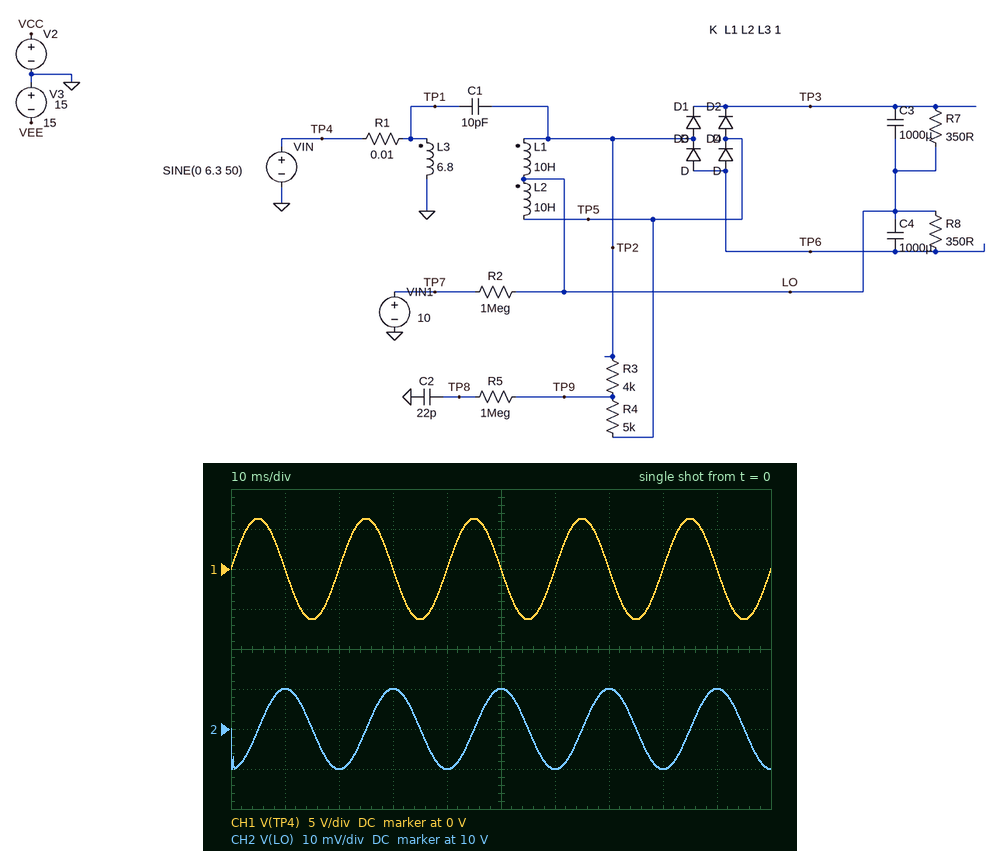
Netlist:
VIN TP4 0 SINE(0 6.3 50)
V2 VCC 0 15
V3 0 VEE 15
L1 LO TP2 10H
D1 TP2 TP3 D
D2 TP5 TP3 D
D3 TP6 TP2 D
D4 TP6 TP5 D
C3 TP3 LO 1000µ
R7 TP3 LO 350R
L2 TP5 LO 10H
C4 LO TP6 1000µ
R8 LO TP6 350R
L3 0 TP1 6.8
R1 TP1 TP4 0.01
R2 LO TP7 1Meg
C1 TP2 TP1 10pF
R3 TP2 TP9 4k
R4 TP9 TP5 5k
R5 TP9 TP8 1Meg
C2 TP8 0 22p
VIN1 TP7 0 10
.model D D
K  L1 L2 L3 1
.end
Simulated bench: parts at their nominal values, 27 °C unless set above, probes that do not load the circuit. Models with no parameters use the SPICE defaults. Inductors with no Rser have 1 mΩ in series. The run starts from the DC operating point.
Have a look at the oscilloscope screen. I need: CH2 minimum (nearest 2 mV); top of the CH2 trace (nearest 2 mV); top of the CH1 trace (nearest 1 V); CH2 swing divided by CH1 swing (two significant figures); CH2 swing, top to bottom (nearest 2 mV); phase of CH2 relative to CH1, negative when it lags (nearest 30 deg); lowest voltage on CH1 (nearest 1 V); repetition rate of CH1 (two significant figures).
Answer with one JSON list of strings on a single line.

["9.990 V", "10.010 V", "6 V", "0.0016", "20 mV", "-90 deg", "-6 V", "50 Hz"]
